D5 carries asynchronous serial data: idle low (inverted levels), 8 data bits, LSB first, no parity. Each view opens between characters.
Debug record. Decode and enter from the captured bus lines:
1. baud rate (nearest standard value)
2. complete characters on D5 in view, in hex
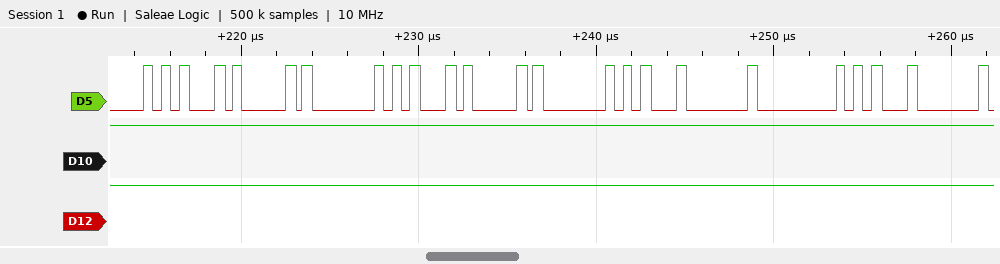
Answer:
2000000 baud
75, 5F, 75, 5F, 75, FF, 75
